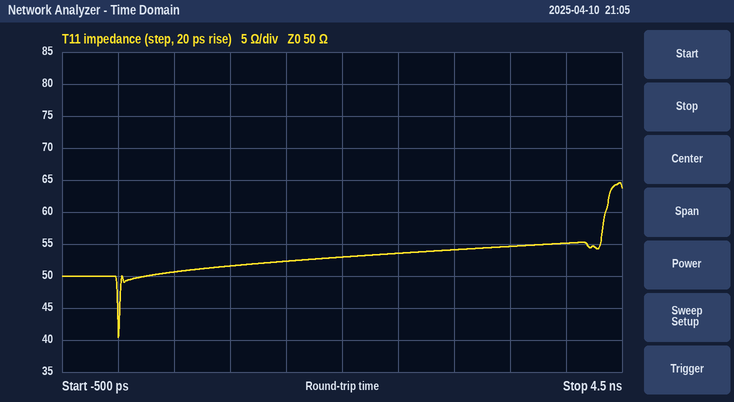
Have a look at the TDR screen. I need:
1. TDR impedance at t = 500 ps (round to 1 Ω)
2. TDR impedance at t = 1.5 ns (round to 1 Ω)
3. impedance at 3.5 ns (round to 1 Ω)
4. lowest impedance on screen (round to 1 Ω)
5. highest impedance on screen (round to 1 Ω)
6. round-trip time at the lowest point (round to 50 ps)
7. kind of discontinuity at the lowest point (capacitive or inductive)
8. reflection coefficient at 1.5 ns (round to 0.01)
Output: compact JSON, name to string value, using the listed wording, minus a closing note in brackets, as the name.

{"TDR impedance at t = 500 ps": "51 Ω", "TDR impedance at t = 1.5 ns": "52 Ω", "impedance at 3.5 ns": "55 Ω", "lowest impedance on screen": "40 Ω", "highest impedance on screen": "65 Ω", "round-trip time at the lowest point": "0 ps", "kind of discontinuity at the lowest point": "capacitive", "reflection coefficient at 1.5 ns": "+0.02"}
